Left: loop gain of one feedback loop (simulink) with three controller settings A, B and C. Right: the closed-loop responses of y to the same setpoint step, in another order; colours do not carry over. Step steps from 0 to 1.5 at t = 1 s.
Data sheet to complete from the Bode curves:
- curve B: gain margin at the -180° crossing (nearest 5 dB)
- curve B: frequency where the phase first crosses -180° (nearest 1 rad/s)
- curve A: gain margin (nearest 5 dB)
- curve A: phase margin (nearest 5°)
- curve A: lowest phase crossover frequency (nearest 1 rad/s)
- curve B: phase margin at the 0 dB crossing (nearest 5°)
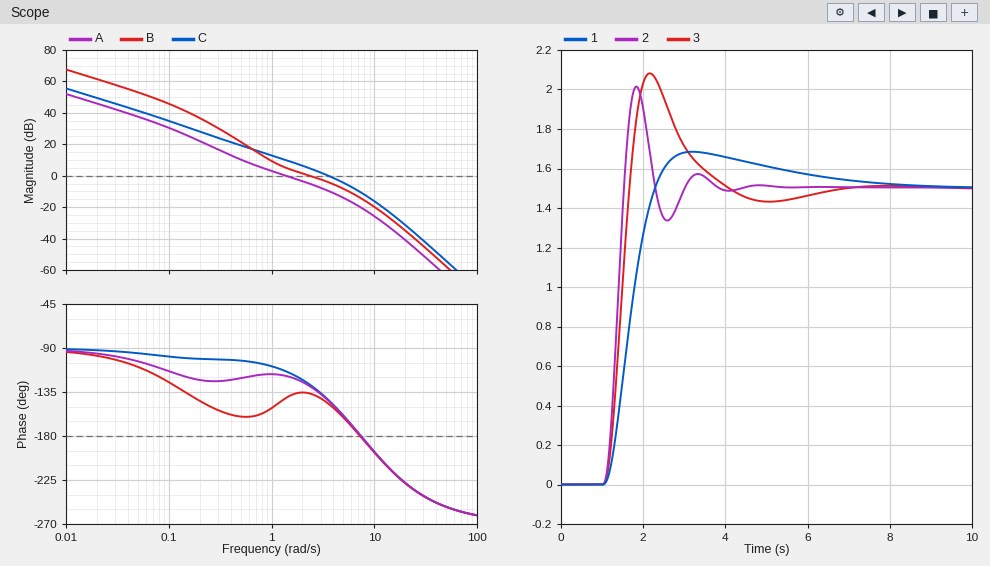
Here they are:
15 dB
7 rad/s
20 dB
60°
7 rad/s
45°
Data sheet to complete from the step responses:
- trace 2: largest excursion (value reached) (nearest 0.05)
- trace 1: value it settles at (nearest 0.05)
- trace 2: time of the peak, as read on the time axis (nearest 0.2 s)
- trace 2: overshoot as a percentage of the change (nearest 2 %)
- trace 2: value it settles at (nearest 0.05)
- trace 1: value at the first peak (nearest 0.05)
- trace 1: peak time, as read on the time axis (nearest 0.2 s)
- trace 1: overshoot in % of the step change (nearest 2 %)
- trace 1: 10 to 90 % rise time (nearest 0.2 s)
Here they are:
2.00
1.50
1.8 s
34 %
1.50
1.70
3.2 s
12 %
0.8 s
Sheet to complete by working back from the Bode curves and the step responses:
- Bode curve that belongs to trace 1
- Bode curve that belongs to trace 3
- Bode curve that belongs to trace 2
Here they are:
A
B
C
